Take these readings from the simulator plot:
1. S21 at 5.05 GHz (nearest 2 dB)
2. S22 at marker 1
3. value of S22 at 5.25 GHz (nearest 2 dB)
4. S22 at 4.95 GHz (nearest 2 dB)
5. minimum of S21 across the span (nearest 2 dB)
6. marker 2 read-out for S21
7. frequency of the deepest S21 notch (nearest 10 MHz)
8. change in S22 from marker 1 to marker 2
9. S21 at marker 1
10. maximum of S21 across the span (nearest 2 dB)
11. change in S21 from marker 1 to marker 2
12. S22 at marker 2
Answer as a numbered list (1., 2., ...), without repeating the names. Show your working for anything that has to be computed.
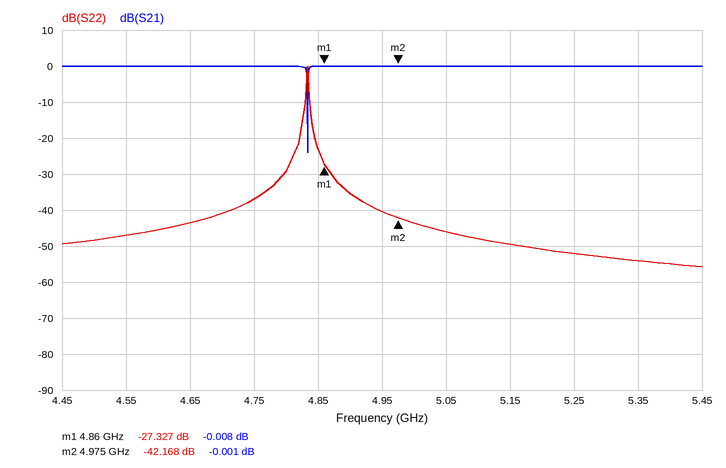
1. 0 dB
2. -27.327 dB
3. -52 dB
4. -40 dB
5. -24 dB
6. -0.001 dB
7. 4.83 GHz
8. -42.168 − (-27.327) = -14.841 dB
9. -0.008 dB
10. 0 dB
11. -0.001 − (-0.008) = 0.007 dB
12. -42.168 dB
